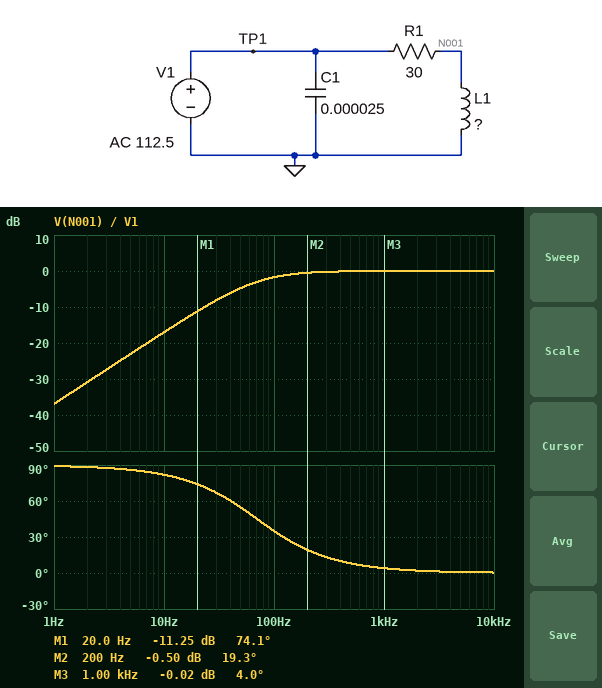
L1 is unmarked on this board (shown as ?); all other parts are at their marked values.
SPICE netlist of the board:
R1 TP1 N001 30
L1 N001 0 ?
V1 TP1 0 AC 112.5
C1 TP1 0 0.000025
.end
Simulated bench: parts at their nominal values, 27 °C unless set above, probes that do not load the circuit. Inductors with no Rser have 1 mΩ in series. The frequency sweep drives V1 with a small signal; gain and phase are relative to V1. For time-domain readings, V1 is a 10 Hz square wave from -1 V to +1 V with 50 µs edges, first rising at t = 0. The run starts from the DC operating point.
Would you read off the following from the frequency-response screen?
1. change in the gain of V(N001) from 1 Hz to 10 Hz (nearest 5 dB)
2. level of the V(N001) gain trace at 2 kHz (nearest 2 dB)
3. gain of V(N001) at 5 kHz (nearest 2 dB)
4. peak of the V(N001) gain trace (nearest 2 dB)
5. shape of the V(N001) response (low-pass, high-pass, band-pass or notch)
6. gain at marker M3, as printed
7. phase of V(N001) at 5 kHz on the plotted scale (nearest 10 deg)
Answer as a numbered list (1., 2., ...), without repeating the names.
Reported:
1. 20 dB
2. 0 dB
3. 0 dB
4. 0 dB
5. high-pass
6. -0.02 dB
7. 0 deg
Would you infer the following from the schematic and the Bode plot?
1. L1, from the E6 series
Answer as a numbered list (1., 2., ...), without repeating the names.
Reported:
1. 68 mH
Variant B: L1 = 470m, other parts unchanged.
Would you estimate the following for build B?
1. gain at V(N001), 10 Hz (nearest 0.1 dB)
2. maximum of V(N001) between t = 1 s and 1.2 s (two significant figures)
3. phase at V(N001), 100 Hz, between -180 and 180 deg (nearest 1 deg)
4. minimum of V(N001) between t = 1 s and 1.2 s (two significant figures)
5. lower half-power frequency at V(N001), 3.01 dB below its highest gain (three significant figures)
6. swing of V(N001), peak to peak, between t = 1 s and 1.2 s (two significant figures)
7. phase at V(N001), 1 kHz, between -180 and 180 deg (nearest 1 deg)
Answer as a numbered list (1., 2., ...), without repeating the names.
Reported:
1. -3.1 dB
2. 1.9 V
3. 6 deg
4. -1.9 V
5. 10.2 Hz
6. 3.8 V
7. 1 deg
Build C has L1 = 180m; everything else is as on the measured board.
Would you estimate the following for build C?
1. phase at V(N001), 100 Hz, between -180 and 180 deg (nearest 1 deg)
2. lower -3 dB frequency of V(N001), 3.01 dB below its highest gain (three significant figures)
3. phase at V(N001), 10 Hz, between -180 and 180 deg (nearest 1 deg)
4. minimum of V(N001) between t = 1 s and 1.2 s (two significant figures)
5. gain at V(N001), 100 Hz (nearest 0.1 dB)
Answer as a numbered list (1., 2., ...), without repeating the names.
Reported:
1. 15 deg
2. 26.5 Hz
3. 69 deg
4. -2.0 V
5. -0.3 dB
